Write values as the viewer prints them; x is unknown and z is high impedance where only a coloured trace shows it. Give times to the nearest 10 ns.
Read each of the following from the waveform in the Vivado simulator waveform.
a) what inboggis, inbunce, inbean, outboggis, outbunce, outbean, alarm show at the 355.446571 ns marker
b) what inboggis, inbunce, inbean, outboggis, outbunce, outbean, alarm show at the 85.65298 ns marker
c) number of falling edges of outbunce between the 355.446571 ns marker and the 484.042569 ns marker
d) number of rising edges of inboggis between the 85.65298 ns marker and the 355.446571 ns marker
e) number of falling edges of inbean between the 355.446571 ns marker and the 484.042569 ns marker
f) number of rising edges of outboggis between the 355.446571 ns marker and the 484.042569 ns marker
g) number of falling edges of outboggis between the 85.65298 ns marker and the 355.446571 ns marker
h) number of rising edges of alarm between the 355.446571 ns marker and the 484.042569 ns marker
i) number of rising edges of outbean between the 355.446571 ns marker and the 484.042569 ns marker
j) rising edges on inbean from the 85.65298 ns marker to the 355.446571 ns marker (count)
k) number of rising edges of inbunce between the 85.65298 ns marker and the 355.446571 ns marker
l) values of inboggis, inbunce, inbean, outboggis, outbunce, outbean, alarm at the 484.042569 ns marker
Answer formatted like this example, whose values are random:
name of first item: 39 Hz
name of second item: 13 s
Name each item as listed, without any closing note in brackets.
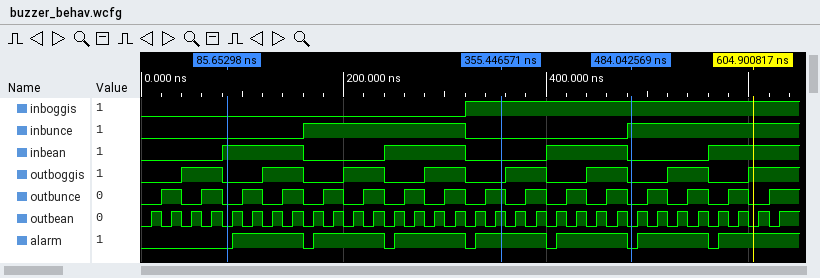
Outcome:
what inboggis, inbunce, inbean, outboggis, outbunce, outbean, alarm show at the 355.446571 ns marker: inboggis=1, inbunce=0, inbean=0, outboggis=0, outbunce=1, outbean=1, alarm=1
what inboggis, inbunce, inbean, outboggis, outbunce, outbean, alarm show at the 85.65298 ns marker: inboggis=0, inbunce=0, inbean=1, outboggis=0, outbunce=0, outbean=0, alarm=0
number of falling edges of outbunce between the 355.446571 ns marker and the 484.042569 ns marker: 4
number of rising edges of inboggis between the 85.65298 ns marker and the 355.446571 ns marker: 1
number of falling edges of inbean between the 355.446571 ns marker and the 484.042569 ns marker: 1
number of rising edges of outboggis between the 355.446571 ns marker and the 484.042569 ns marker: 2
number of falling edges of outboggis between the 85.65298 ns marker and the 355.446571 ns marker: 3
number of rising edges of alarm between the 355.446571 ns marker and the 484.042569 ns marker: 1
number of rising edges of outbean between the 355.446571 ns marker and the 484.042569 ns marker: 6
rising edges on inbean from the 85.65298 ns marker to the 355.446571 ns marker: 1
number of rising edges of inbunce between the 85.65298 ns marker and the 355.446571 ns marker: 1
values of inboggis, inbunce, inbean, outboggis, outbunce, outbean, alarm at the 484.042569 ns marker: inboggis=1, inbunce=1, inbean=0, outboggis=0, outbunce=0, outbean=0, alarm=0
